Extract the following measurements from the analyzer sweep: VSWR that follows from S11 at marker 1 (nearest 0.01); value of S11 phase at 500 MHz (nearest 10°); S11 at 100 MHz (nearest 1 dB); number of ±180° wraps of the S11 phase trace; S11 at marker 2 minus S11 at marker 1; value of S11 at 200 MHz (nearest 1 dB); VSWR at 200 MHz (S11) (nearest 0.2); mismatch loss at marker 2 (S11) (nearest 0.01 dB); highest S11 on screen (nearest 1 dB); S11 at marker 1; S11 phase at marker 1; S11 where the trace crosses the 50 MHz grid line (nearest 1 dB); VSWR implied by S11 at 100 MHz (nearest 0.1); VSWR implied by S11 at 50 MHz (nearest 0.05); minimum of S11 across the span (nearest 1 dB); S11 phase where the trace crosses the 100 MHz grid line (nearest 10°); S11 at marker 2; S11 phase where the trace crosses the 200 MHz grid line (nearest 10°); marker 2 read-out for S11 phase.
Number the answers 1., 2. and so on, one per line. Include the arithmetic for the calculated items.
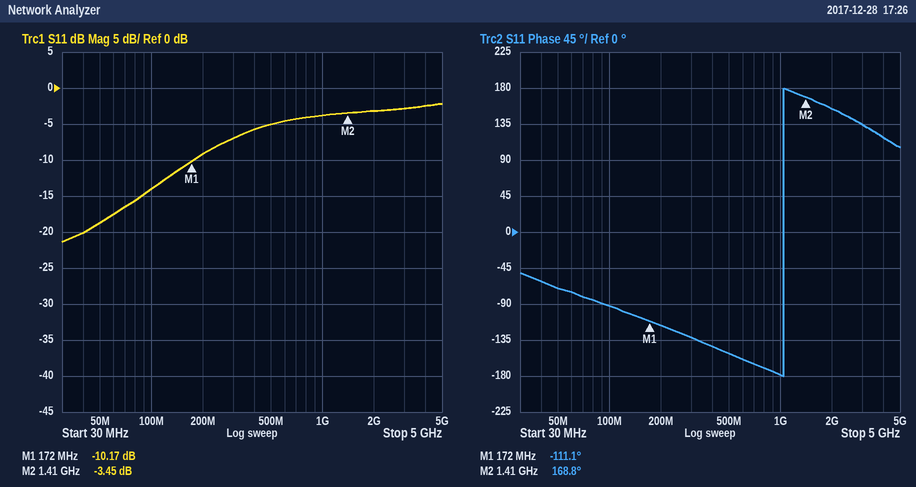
1. (1 + 0.3101)/(1 − 0.3101) ≈ 1.90
2. -150°
3. -14 dB
4. 1
5. -3.45 − (-10.17) = 6.72 dB
6. -9 dB
7. |Γ| = 10^(-9/20) = 0.3548; VSWR = (1 + 0.3548)/(1 − 0.3548) ≈ 2.10, so 2.0 to the nearest 0.2
8. −10 log10(1 − 10^(-3.45/10)) ≈ 2.61 dB
9. -2 dB
10. -10.17 dB
11. -111.1°
12. -19 dB
13. |Γ| = 10^(-14/20) = 0.1995; VSWR = (1 + 0.1995)/(1 − 0.1995) ≈ 1.5
14. |Γ| = 10^(-19/20) = 0.1122; VSWR = (1 + 0.1122)/(1 − 0.1122) ≈ 1.25
15. -21 dB
16. -90°
17. -3.45 dB
18. -120°
19. 168.8°
